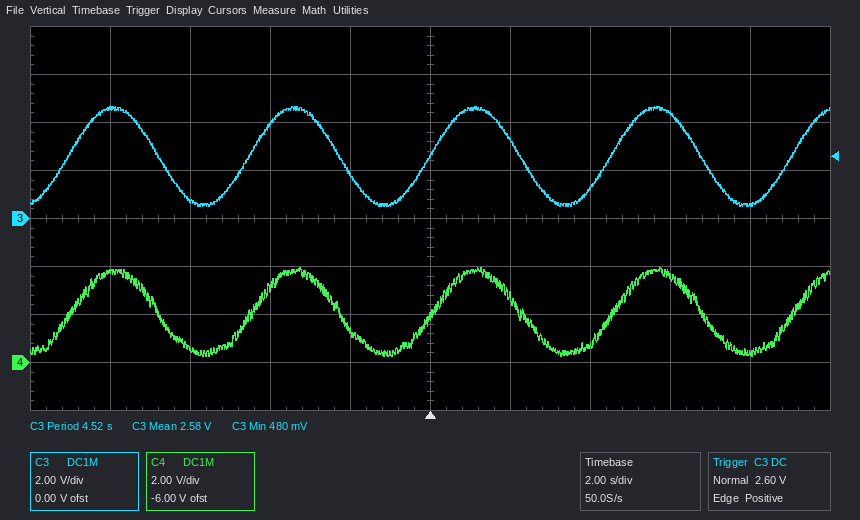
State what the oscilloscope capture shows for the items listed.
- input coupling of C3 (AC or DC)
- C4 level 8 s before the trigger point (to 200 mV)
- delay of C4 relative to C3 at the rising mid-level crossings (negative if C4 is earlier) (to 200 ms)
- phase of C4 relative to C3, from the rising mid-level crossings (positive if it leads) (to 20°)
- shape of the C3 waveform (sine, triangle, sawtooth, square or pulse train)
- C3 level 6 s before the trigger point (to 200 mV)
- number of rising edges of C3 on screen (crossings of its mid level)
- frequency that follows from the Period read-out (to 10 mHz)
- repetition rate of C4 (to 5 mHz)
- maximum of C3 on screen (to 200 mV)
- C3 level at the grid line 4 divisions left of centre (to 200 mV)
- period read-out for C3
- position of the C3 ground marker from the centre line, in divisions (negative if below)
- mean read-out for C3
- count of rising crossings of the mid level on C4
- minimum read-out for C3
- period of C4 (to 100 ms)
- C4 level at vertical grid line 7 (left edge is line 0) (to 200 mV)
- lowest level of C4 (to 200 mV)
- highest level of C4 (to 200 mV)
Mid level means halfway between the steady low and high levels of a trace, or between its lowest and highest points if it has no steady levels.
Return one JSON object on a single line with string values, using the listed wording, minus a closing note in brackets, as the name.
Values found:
{"input coupling of C3": "DC", "C4 level 8 s before the trigger point": "3.8 V", "delay of C4 relative to C3 at the rising mid-level crossings (negative if C4 is earlier)": "0.0 s", "phase of C4 relative to C3, from the rising mid-level crossings (positive if it leads)": "0°", "shape of the C3 waveform": "sine", "C3 level 6 s before the trigger point": "800 mV", "number of rising edges of C3 on screen": "5", "frequency that follows from the Period read-out": "220 mHz", "repetition rate of C4": "220 mHz", "maximum of C3 on screen": "4.6 V", "C3 level at the grid line 4 divisions left of centre": "4.6 V", "period read-out for C3": "4.52 s", "position of the C3 ground marker from the centre line, in divisions": "0.0 div", "mean read-out for C3": "2.58 V", "count of rising crossings of the mid level on C4": "5", "minimum read-out for C3": "480 mV", "period of C4": "4.5 s", "C4 level at vertical grid line 7 (left edge is line 0)": "800 mV", "lowest level of C4": "200 mV", "highest level of C4": "4.0 V"}
